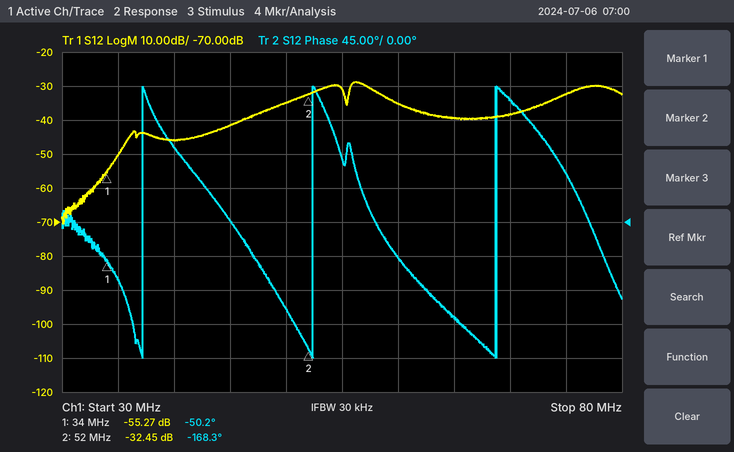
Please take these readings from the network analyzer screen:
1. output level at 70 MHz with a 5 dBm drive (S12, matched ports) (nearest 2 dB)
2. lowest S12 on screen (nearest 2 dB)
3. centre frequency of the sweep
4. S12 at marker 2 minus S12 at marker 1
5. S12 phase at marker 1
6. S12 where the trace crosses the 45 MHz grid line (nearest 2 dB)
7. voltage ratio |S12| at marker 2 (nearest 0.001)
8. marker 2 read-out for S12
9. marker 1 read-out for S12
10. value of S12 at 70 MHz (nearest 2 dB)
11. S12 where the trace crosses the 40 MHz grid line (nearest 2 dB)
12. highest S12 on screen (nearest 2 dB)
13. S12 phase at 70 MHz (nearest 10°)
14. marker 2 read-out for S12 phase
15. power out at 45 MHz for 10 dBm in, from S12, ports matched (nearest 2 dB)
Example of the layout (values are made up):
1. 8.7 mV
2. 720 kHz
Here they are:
1. -34 dBm
2. -70 dB
3. 55 MHz
4. 22.82 dB
5. -50.2°
6. -42 dB
7. 0.024
8. -32.45 dB
9. -55.27 dB
10. -38 dB
11. -46 dB
12. -28 dB
13. 160°
14. -168.3°
15. -32 dBm
